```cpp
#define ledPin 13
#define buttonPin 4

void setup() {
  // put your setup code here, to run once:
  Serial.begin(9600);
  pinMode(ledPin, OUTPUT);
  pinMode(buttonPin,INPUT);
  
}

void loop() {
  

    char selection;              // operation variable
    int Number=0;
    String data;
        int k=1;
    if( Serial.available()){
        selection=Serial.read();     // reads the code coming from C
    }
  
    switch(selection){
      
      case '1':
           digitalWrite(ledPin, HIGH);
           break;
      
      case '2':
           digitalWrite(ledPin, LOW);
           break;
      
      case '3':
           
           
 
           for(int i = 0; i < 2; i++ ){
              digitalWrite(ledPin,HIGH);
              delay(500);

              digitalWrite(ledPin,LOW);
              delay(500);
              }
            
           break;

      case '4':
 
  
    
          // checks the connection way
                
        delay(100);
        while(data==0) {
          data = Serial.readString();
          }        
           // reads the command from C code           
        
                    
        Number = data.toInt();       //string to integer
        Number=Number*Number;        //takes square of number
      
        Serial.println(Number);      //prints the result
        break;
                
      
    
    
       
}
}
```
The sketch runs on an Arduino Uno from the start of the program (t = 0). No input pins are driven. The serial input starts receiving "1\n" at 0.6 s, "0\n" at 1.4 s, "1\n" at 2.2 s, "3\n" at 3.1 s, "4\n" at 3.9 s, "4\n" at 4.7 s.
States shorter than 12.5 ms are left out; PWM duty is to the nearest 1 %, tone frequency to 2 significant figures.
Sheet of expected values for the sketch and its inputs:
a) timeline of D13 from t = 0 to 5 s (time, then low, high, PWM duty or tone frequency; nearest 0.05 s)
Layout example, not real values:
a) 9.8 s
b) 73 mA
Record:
a) 0 s low; 0.6 s high; 3.6 s low; 4.1 s high; 4.6 s low
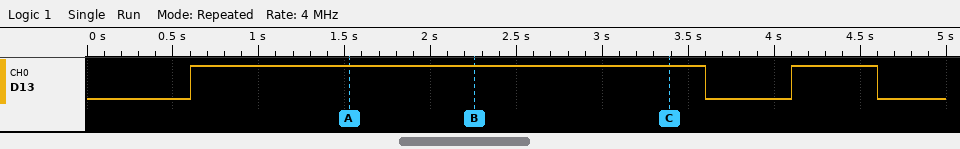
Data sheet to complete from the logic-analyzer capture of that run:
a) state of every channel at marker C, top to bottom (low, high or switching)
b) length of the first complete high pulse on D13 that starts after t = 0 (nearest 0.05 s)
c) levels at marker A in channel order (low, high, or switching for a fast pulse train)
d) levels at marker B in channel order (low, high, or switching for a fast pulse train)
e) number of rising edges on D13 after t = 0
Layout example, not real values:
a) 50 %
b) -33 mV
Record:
a) D13 high
b) 3.00 s
c) D13 high
d) D13 high
e) 2
